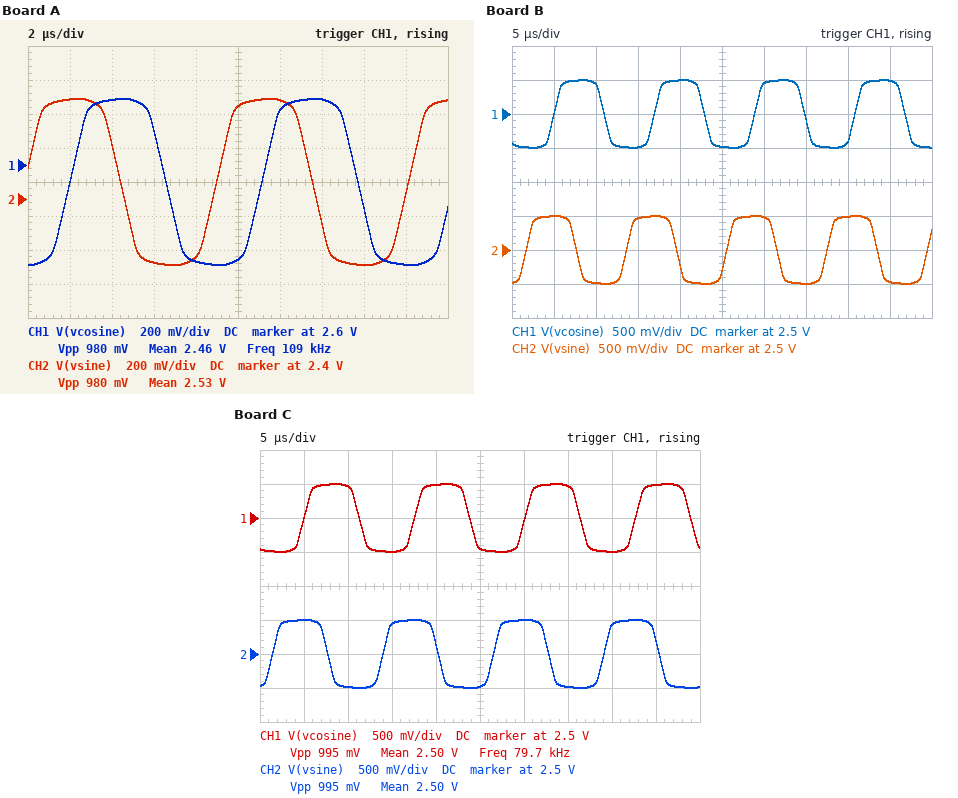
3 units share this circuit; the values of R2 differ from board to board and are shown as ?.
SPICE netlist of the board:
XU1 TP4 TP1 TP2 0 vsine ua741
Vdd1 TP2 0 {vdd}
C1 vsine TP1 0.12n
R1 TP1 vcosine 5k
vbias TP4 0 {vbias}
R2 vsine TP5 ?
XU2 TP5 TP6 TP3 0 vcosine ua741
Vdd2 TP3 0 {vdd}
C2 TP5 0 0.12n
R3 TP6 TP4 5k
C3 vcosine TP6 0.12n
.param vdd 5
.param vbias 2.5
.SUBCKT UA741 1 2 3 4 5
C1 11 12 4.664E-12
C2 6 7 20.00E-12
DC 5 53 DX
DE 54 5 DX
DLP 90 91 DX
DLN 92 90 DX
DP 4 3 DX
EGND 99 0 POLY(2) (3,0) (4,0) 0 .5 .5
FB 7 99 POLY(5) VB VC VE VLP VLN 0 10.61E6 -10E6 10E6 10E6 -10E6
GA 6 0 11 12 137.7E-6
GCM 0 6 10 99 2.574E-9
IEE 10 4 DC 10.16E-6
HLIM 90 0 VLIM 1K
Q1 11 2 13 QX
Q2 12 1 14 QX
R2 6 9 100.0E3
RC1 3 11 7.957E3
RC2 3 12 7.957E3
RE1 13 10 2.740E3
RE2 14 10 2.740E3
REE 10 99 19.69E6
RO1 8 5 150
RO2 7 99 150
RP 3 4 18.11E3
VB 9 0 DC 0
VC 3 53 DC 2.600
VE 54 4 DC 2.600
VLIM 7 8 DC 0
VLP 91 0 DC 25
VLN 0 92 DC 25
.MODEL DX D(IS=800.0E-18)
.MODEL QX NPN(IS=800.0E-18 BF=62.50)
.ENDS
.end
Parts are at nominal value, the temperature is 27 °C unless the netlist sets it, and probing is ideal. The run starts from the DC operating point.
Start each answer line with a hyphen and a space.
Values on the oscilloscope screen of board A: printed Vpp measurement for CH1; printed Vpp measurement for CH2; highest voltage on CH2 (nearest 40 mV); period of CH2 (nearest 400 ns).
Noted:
- 980 mV
- 980 mV
- 3.00 V
- 9.2 µs
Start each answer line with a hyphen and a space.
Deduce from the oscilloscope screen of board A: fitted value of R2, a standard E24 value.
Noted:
- 2.4 kΩ
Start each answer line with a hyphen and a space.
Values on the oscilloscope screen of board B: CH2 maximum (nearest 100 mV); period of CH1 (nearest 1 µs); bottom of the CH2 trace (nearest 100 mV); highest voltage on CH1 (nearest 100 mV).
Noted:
- 3.0 V
- 12 µs
- 2.0 V
- 3.0 V
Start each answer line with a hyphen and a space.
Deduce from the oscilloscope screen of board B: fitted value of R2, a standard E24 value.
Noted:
- 13 kΩ
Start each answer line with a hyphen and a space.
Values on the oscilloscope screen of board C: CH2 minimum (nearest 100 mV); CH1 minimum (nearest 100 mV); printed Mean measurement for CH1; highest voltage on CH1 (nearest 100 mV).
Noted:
- 2.0 V
- 2.0 V
- 2.50 V
- 3.0 V
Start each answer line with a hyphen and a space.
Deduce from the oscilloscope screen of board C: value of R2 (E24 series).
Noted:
- 16 kΩ
